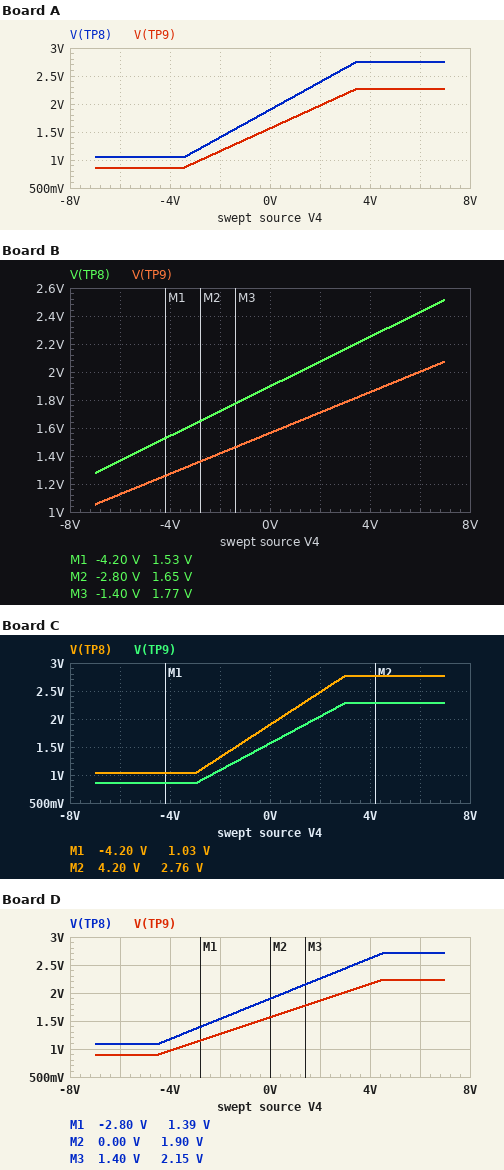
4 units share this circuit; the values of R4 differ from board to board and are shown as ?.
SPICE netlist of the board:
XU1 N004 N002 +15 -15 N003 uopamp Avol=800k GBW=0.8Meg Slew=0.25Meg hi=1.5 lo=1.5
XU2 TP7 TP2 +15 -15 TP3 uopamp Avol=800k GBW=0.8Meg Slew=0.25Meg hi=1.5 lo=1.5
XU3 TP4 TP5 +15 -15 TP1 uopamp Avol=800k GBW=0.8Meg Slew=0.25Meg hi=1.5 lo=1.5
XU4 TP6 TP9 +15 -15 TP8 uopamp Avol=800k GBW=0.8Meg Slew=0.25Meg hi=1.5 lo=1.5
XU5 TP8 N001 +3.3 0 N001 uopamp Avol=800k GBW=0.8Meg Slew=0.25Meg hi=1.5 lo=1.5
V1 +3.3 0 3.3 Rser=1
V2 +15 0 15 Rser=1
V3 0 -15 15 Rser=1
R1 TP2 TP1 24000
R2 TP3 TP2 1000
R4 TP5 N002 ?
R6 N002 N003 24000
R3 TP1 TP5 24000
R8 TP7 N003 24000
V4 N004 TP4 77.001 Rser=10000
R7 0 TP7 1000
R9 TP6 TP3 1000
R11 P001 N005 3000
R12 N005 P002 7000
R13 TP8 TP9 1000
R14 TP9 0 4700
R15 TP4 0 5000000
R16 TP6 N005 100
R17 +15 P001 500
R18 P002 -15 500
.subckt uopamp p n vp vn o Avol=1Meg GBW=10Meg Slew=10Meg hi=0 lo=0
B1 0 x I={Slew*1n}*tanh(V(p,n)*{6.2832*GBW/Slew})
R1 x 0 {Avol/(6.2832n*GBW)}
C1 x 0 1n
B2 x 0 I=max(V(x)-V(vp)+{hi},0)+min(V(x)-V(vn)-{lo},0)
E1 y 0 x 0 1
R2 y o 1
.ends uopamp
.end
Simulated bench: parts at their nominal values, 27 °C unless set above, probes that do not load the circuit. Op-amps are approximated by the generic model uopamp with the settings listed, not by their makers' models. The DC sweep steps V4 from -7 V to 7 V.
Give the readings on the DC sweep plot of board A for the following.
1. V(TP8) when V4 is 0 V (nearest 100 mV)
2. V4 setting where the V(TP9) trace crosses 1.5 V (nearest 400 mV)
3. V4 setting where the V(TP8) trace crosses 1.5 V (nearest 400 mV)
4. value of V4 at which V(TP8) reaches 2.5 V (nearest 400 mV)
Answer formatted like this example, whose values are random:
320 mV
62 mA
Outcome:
1.9 V
-400 mV
-1.6 V
2.4 V
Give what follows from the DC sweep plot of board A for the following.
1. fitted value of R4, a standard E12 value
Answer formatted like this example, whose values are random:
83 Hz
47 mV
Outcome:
8.2 kΩ
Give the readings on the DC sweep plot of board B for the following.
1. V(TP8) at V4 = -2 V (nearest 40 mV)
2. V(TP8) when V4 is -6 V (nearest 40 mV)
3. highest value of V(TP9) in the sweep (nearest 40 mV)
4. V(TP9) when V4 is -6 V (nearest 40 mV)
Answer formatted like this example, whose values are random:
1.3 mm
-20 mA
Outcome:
1.72 V
1.36 V
2.08 V
1.12 V
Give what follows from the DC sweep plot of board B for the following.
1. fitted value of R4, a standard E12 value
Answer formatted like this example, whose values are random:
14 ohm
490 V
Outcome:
33 kΩ
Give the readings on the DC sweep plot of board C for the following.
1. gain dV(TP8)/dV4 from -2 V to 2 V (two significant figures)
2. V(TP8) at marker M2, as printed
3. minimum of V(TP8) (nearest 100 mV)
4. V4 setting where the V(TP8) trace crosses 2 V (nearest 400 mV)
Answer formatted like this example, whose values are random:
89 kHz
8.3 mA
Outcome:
0.29 V/V
2.76 V
1.0 V
400 mV
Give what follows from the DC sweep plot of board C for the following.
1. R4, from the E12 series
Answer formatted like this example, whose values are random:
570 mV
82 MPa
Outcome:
6.8 kΩ
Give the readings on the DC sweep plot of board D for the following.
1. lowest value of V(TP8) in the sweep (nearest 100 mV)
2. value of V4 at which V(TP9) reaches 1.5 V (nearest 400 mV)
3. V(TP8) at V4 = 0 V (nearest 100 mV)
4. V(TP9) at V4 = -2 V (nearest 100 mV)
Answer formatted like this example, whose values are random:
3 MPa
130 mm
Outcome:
1.1 V
-400 mV
1.9 V
1.3 V
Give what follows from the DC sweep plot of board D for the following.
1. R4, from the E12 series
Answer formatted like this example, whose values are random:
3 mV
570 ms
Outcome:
12 kΩ
